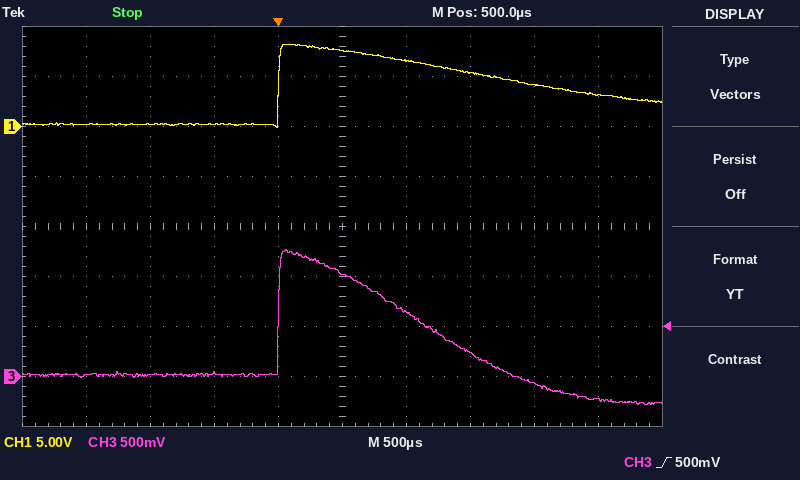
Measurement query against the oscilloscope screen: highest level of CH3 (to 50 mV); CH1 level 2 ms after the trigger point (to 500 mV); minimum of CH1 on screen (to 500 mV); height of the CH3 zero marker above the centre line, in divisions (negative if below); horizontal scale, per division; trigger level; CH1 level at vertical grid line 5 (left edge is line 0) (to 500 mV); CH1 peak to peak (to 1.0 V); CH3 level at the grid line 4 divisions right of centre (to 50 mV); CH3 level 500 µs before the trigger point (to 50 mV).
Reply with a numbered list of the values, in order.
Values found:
1. 1.25 V
2. 4.0 V
3. 0.0 V
4. -3.0 div
5. 500 µs
6. 500 mV
7. 7.5 V
8. 8.0 V
9. -250 mV
10. 50 mV
